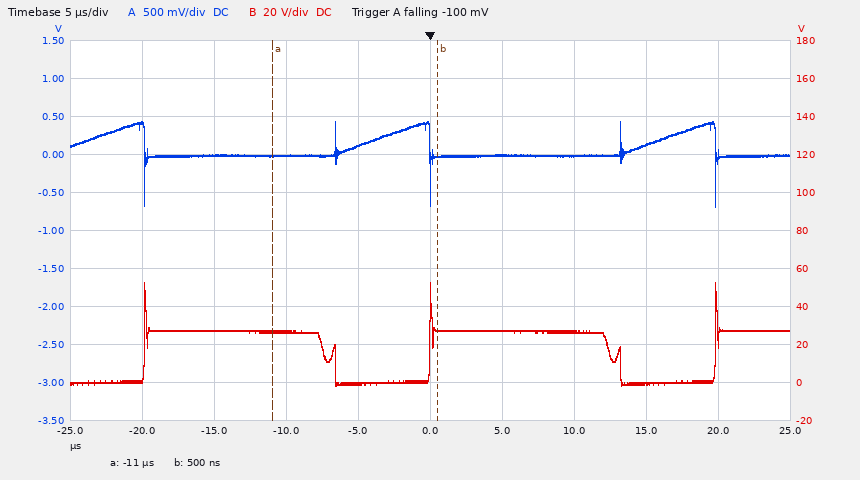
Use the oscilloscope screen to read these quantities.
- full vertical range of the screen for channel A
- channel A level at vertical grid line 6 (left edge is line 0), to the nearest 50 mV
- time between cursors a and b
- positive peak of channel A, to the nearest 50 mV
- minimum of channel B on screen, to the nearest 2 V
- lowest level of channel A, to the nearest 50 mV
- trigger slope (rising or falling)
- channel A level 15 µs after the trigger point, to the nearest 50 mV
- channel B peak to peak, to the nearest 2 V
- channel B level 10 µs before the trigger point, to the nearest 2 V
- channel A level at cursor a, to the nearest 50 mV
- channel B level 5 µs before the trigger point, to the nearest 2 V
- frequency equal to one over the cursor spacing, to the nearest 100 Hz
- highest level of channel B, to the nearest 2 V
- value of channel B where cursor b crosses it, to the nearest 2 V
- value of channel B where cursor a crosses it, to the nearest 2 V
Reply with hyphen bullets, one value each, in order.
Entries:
- 5 V
- 0 mV
- 11.5 µs
- 450 mV
- -2 V
- -700 mV
- falling
- 150 mV
- 54 V
- 26 V
- 0 mV
- 0 V
- 87.0 kHz
- 52 V
- 28 V
- 26 V
